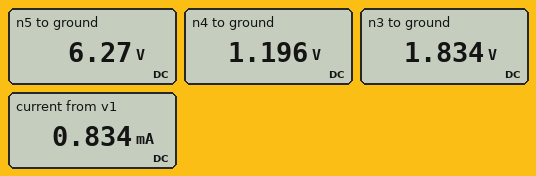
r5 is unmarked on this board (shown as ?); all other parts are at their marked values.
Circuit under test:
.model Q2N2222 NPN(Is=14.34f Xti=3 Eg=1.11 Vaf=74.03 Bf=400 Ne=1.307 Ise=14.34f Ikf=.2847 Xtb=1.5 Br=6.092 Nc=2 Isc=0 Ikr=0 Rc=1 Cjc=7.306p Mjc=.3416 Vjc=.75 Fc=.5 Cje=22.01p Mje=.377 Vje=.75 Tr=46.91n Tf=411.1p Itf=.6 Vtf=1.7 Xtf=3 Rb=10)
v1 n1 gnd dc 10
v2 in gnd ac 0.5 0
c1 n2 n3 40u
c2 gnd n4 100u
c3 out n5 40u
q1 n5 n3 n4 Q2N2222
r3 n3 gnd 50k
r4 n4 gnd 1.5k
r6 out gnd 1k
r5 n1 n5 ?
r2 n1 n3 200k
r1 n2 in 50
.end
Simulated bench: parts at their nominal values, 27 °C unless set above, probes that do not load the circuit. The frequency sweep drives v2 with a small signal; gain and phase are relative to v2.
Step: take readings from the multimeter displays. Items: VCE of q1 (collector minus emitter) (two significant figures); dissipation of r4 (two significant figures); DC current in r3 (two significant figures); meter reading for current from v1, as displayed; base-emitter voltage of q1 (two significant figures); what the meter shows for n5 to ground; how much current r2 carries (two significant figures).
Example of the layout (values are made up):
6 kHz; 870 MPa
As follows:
5.1 V; 950 µW; 37 µA; 0.834 mA; 640 mV; 6.27 V; 41 µA
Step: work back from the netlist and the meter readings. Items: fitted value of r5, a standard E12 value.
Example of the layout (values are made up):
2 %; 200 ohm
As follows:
4.7 kΩ
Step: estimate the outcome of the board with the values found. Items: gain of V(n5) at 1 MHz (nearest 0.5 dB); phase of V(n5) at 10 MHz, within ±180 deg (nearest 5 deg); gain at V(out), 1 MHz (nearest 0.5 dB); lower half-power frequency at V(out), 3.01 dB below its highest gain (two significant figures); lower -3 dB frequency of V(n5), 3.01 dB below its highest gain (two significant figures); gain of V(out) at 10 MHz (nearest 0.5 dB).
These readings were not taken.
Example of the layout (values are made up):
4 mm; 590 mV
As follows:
28.0 dB; 140 deg; 28.0 dB; 50 Hz; 49 Hz; 26.0 dB
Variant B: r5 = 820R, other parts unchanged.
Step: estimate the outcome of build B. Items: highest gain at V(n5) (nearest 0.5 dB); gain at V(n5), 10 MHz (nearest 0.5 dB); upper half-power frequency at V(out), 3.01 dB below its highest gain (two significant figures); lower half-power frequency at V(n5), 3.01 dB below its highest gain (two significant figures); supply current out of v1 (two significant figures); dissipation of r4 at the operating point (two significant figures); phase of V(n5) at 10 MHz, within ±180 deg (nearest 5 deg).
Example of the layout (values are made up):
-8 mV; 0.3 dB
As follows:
22.5 dB; 22.0 dB; 24 MHz; 50 Hz; 840 µA; 960 µW; 155 deg
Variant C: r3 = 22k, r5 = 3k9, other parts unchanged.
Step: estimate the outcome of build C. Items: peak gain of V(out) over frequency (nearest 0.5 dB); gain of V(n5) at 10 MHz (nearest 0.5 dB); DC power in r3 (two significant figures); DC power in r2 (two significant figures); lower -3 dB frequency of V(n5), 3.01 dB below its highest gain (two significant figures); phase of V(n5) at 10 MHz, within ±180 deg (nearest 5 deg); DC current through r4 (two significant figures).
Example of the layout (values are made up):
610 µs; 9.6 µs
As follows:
17.0 dB; 16.5 dB; 42 µW; 410 µW; 15 Hz; 155 deg; 240 µA
